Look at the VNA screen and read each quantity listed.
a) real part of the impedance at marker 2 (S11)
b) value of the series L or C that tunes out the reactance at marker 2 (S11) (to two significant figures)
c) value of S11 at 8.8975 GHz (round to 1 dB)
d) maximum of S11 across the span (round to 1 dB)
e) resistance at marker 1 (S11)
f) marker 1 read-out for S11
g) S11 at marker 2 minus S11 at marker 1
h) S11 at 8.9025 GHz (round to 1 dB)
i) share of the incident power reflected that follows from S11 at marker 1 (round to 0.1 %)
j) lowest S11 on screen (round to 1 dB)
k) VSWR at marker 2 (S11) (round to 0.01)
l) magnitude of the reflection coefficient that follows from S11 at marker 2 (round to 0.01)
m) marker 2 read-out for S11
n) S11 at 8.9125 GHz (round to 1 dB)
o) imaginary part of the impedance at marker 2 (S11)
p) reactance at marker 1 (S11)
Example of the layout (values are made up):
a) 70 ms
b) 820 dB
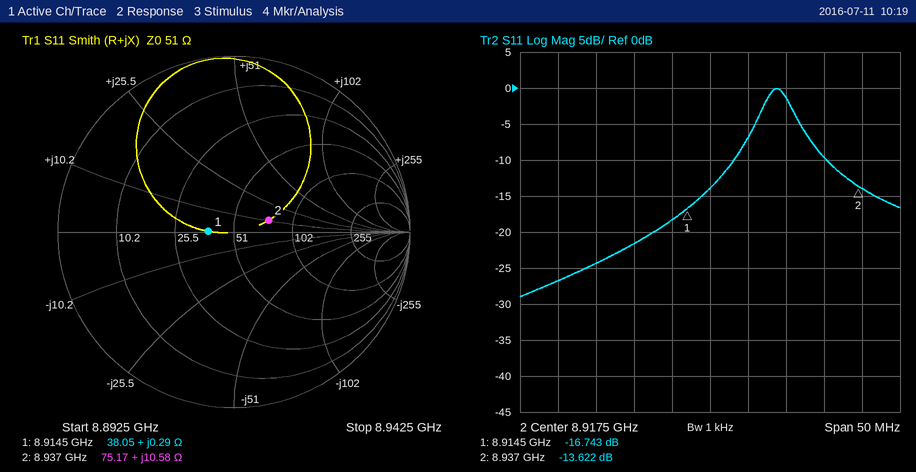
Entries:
a) 75.17 Ω
b) 1.7 pF
c) -27 dB
d) 0 dB
e) 38.05 Ω
f) -16.743 dB
g) 3.121 dB
h) -24 dB
i) 2.1 %
j) -29 dB
k) 1.53
l) 0.21
m) -13.622 dB
n) -18 dB
o) +10.58 Ω
p) +0.29 Ω
